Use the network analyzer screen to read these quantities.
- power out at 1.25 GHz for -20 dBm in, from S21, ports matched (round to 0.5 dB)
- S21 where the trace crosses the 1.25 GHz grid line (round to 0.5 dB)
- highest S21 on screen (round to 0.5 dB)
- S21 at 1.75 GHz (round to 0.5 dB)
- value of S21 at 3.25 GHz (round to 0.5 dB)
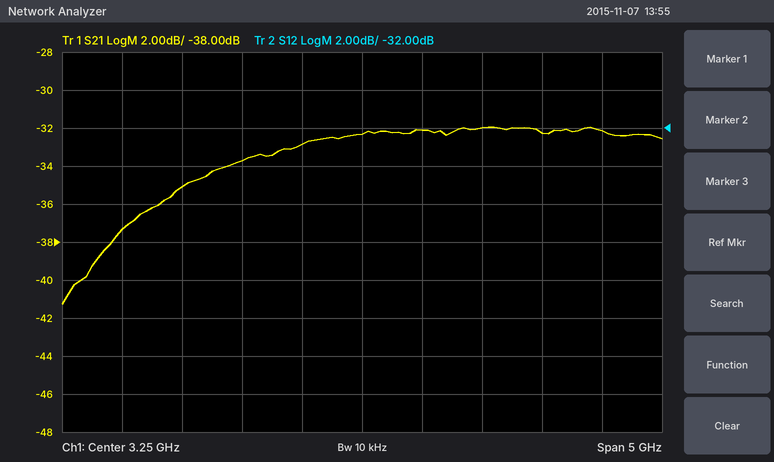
-57.5 dBm
-37.5 dB
-32.0 dB
-35.0 dB
-32.5 dB
